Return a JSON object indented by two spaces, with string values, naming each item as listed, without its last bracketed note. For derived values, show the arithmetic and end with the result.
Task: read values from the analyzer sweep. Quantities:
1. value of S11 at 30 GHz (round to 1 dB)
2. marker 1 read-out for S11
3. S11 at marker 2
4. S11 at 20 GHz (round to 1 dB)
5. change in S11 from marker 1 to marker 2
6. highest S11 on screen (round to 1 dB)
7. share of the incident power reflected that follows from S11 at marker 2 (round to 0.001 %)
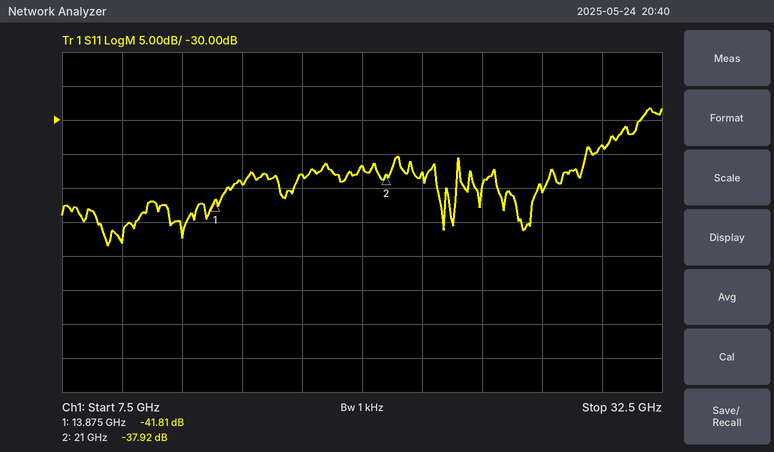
{
  "value of S11 at 30 GHz": "-34 dB",
  "marker 1 read-out for S11": "-41.81 dB",
  "S11 at marker 2": "-37.92 dB",
  "S11 at 20 GHz": "-37 dB",
  "change in S11 from marker 1 to marker 2": "-37.92 − (-41.81) = 3.89 dB",
  "highest S11 on screen": "-28 dB",
  "share of the incident power reflected that follows from S11 at marker 2": "10^(-37.92/10) ≈ 0.016 %"
}
